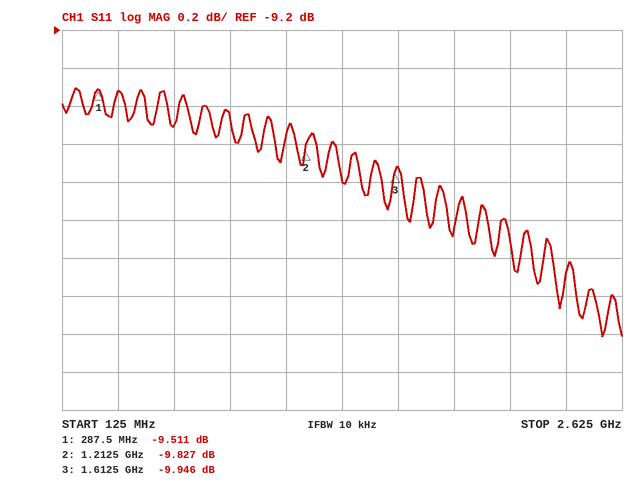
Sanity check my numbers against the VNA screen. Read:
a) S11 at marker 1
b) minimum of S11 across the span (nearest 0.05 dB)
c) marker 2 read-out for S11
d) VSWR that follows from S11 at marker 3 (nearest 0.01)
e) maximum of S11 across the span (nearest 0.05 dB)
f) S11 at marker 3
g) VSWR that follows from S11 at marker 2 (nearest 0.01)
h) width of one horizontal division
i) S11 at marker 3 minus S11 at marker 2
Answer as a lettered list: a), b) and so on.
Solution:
a) -9.511 dB
b) -10.80 dB
c) -9.827 dB
d) 1.93
e) -9.50 dB
f) -9.946 dB
g) 1.95
h) 250 MHz
i) -0.119 dB
